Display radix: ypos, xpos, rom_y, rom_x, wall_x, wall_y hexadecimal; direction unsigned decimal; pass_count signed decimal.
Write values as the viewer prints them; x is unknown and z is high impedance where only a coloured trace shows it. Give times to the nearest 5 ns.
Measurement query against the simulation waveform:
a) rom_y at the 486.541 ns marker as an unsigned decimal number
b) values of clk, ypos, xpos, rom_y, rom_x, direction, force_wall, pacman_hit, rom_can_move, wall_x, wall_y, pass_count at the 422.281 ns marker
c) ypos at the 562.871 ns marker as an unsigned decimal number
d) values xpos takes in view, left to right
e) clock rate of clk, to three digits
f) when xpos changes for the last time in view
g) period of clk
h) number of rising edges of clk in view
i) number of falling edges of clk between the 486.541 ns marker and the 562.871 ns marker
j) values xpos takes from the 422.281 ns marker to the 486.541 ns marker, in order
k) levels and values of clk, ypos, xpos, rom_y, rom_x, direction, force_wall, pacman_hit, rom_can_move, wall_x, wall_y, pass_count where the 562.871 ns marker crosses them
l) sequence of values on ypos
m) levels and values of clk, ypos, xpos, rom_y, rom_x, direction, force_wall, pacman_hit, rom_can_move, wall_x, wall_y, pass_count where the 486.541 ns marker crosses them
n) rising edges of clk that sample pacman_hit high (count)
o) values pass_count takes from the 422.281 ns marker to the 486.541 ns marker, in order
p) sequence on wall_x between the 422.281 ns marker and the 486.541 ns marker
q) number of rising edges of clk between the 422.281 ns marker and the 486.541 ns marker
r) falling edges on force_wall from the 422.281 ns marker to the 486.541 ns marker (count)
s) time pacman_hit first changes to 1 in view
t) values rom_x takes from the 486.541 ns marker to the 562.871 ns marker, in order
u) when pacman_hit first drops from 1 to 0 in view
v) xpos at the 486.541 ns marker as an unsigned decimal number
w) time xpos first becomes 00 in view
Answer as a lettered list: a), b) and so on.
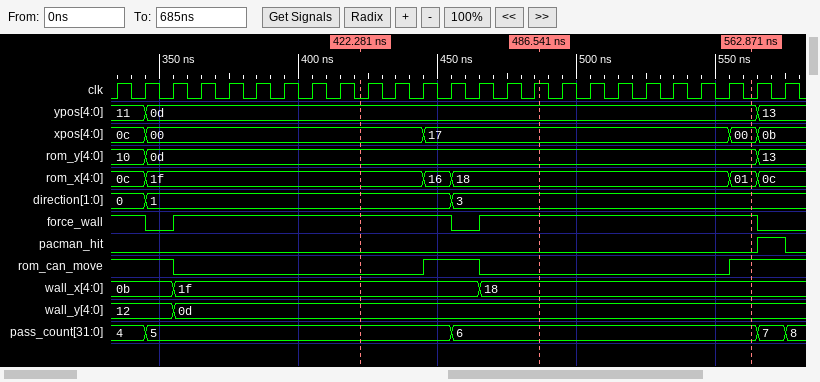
a) 13
b) clk=0, ypos=0d, xpos=00, rom_y=0d, rom_x=1f, direction=1, force_wall=1, pacman_hit=0, rom_can_move=0, wall_x=1f, wall_y=0d, pass_count=5
c) 13
d) 0c, 00, 17, 00, 0b
e) 100 MHz
f) 565 ns
g) 10 ns
h) 25
i) 8
j) 00, 17
k) clk=0, ypos=0d, xpos=00, rom_y=0d, rom_x=01, direction=3, force_wall=1, pacman_hit=0, rom_can_move=1, wall_x=18, wall_y=0d, pass_count=6
l) 11, 0d, 13
m) clk=1, ypos=0d, xpos=17, rom_y=0d, rom_x=18, direction=3, force_wall=1, pacman_hit=0, rom_can_move=0, wall_x=18, wall_y=0d, pass_count=6
n) 1
o) 5, 6
p) 1f, 18
q) 7
r) 1
s) 565 ns
t) 18, 01
u) 575 ns
v) 23
w) 345 ns
